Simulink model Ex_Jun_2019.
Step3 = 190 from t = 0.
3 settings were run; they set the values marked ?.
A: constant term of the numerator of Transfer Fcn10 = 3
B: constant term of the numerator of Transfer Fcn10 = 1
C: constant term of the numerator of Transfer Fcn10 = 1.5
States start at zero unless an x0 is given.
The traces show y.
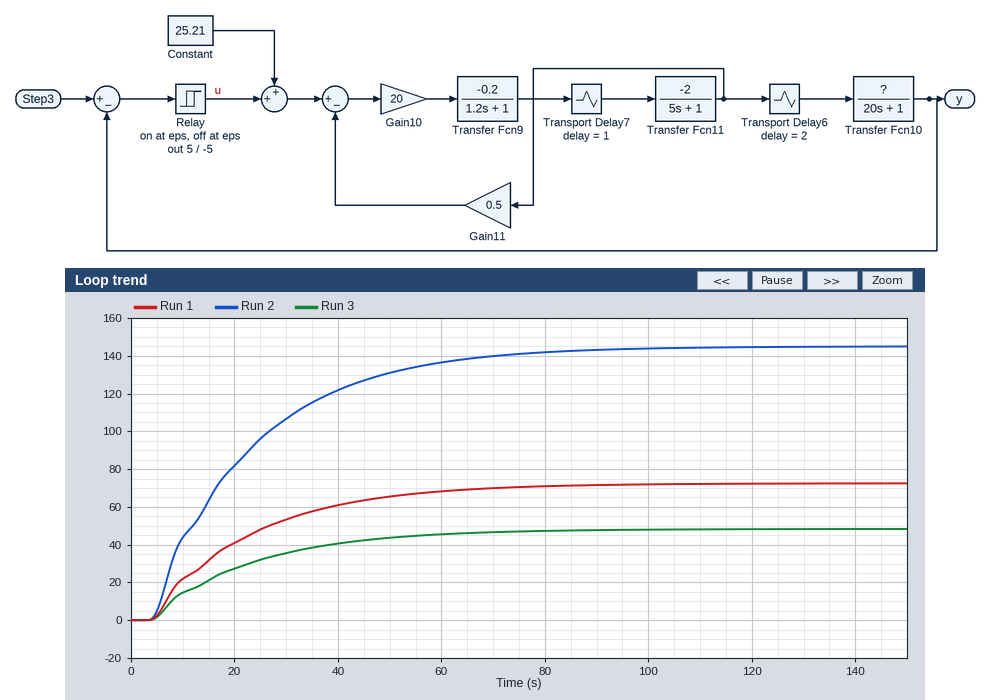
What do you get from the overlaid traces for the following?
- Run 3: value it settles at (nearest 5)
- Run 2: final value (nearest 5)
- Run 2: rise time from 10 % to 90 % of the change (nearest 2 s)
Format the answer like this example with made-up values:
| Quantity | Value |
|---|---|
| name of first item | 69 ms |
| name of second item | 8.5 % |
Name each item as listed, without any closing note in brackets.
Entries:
| Quantity | Value |
|---|---|
| Run 3: value it settles at | 50 |
| Run 2: final value | 145 |
| Run 2: rise time from 10 % to 90 % of the change | 44 s |
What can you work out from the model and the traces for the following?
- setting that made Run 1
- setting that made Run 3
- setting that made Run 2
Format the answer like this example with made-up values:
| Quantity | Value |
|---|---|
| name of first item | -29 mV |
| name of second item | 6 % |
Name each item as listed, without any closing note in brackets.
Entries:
| Quantity | Value |
|---|---|
| setting that made Run 1 | C |
| setting that made Run 3 | B |
| setting that made Run 2 | A |
